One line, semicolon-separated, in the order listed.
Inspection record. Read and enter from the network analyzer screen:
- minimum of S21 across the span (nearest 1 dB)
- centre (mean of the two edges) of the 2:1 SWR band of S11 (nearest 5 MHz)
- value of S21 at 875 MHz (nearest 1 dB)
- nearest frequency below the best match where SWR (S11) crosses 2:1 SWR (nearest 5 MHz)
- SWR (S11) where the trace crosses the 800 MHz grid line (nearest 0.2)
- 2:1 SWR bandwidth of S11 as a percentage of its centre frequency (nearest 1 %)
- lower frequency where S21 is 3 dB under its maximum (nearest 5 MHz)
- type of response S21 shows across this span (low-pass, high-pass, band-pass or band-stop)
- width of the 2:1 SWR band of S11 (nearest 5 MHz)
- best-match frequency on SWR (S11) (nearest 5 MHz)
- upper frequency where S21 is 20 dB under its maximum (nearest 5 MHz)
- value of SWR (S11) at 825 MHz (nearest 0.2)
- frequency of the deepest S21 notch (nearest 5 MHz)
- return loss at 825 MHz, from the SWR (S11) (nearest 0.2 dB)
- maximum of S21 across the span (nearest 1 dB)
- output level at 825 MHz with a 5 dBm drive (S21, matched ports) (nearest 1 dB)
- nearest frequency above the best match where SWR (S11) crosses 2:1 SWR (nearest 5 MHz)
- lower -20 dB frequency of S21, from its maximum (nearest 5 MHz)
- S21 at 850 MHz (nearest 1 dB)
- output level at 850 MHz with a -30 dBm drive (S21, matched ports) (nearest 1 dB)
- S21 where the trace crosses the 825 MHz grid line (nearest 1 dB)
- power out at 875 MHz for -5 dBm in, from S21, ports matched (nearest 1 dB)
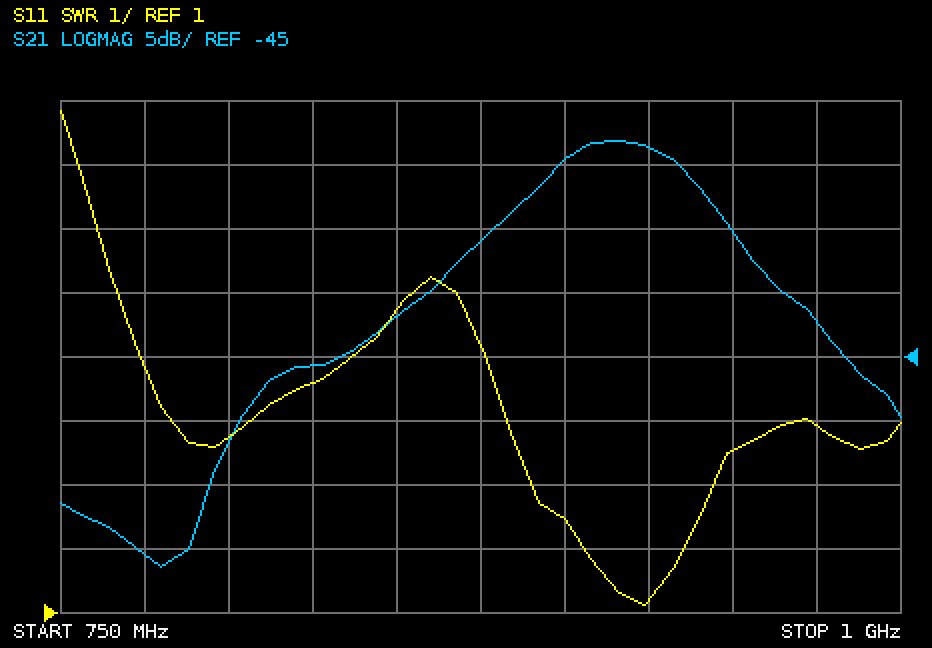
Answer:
-61 dB; 920 MHz; -36 dB; 905 MHz; 3.8; 3 %; 895 MHz; band-pass; 30 MHz; 925 MHz; 995 MHz; 4.6; 780 MHz; 3.8 dB; -28 dB; -41 dBm; 935 MHz; 810 MHz; -42 dB; -72 dBm; -46 dB; -41 dBm
